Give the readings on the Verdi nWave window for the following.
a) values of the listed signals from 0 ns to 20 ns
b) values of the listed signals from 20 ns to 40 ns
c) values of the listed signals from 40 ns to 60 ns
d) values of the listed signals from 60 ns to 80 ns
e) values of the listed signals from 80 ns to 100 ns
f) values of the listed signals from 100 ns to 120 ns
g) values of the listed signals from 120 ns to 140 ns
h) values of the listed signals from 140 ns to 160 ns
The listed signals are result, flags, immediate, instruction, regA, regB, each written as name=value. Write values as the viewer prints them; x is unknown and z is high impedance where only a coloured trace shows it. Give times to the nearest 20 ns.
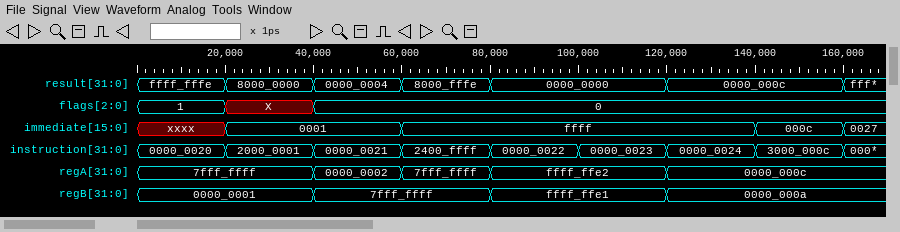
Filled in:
result=ffff_fffe, flags=1, immediate=xxxx, instruction=0000_0020, regA=7fff_ffff, regB=0000_0001
result=8000_0000, flags=X, immediate=0001, instruction=2000_0001, regA=7fff_ffff, regB=0000_0001
result=0000_0004, flags=0, immediate=0001, instruction=0000_0021, regA=0000_0002, regB=7fff_ffff
result=8000_fffe, flags=0, immediate=ffff, instruction=2400_ffff, regA=7fff_ffff, regB=7fff_ffff
result=0000_0000, flags=0, immediate=ffff, instruction=0000_0022, regA=ffff_ffe2, regB=ffff_ffe1
result=0000_0000, flags=0, immediate=ffff, instruction=0000_0023, regA=ffff_ffe2, regB=ffff_ffe1
result=0000_000c, flags=0, immediate=ffff, instruction=0000_0024, regA=0000_000c, regB=0000_000a
result=0000_000c, flags=0, immediate=000c, instruction=3000_000c, regA=0000_000c, regB=0000_000a
